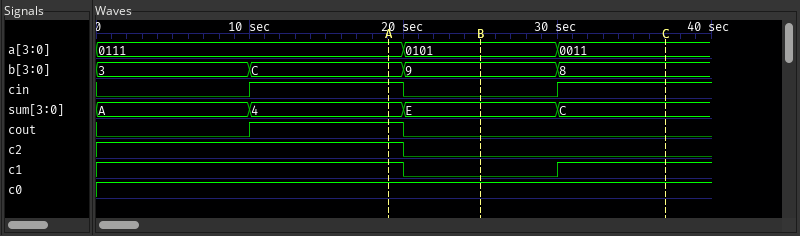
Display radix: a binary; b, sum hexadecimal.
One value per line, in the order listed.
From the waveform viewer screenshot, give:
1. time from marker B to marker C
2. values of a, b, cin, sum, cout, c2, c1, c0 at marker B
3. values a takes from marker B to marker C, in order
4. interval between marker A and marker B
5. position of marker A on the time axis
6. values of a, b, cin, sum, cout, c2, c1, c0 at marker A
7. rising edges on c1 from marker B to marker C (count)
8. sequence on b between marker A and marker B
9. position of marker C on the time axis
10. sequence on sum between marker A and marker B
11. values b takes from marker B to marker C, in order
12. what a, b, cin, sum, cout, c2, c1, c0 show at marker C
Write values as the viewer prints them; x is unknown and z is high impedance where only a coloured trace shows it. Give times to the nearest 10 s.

10 s
a=0101, b=9, cin=0, sum=E, cout=0, c2=0, c1=0, c0=1
0101, 0011
10 s
20 s
a=0111, b=C, cin=1, sum=4, cout=1, c2=1, c1=1, c0=1
1
C, 9
40 s
4, E
9, 8
a=0011, b=8, cin=1, sum=C, cout=0, c2=0, c1=1, c0=1
